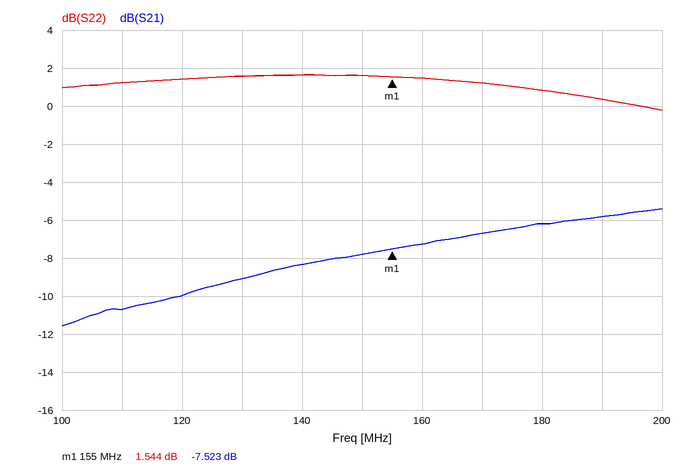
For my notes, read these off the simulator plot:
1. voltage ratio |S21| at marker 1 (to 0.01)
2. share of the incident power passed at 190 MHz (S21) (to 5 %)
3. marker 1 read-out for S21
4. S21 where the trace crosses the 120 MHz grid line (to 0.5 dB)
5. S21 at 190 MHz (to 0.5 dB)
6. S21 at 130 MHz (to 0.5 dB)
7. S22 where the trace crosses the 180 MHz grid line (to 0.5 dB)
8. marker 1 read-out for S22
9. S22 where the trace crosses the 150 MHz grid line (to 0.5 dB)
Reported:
0.42
25 %
-7.523 dB
-10.0 dB
-6.0 dB
-9.0 dB
1.0 dB
1.544 dB
1.5 dB
